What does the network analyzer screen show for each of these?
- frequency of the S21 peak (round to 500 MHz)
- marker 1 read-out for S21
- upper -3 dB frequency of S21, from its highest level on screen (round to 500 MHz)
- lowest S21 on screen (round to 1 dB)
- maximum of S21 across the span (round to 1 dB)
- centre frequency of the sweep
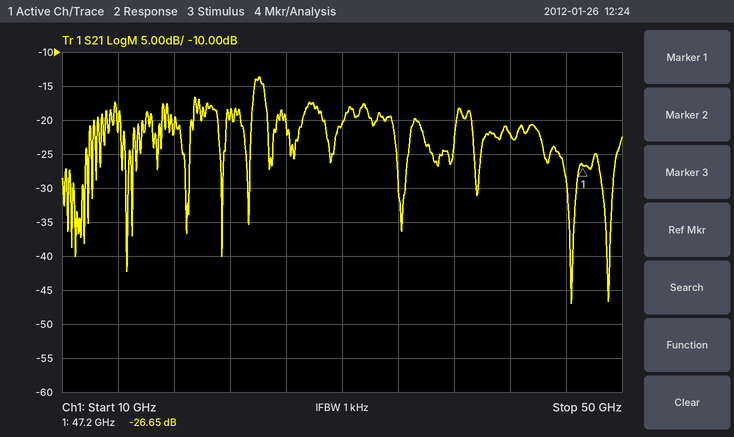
24.0 GHz
-26.65 dB
24.5 GHz
-47 dB
-14 dB
30 GHz
